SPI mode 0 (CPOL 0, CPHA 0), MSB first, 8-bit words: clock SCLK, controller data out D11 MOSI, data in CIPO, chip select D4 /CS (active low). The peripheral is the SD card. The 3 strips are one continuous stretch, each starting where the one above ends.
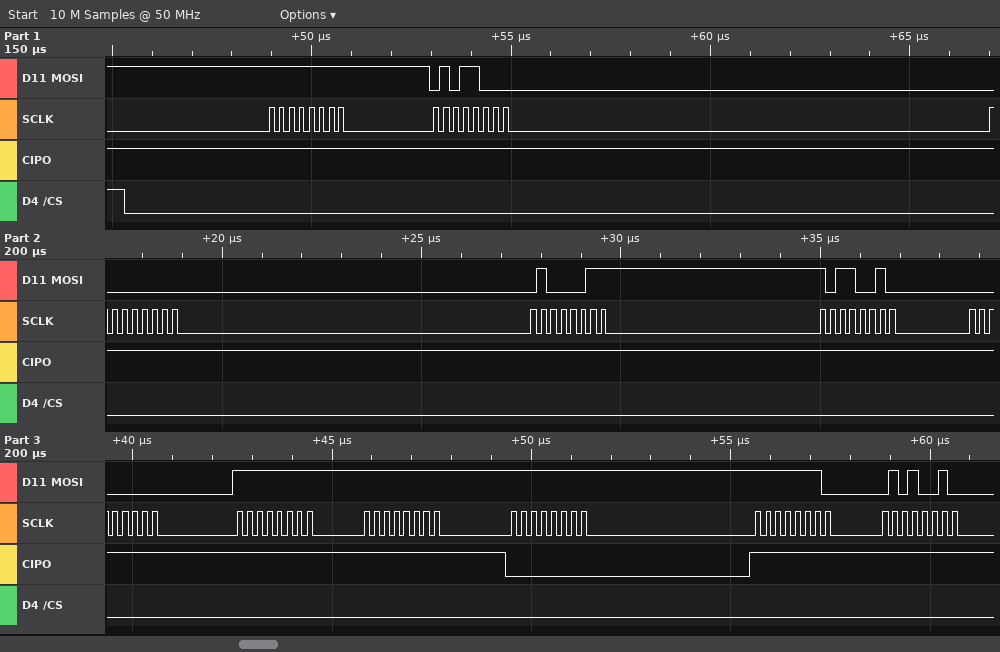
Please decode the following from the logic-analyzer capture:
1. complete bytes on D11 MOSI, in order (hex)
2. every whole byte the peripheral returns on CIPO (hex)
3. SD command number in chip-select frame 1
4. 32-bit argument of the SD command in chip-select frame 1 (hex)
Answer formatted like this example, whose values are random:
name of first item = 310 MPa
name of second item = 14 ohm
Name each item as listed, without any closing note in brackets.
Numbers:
complete bytes on D11 MOSI, in order = FF 58 00 43 B2 00 FF FF FF FE 52
every whole byte the peripheral returns on CIPO = FF FF FF FF FF FF FF FF 00 FF FF
SD command number in chip-select frame 1 = CMD24
32-bit argument of the SD command in chip-select frame 1 = 0x0043B200
